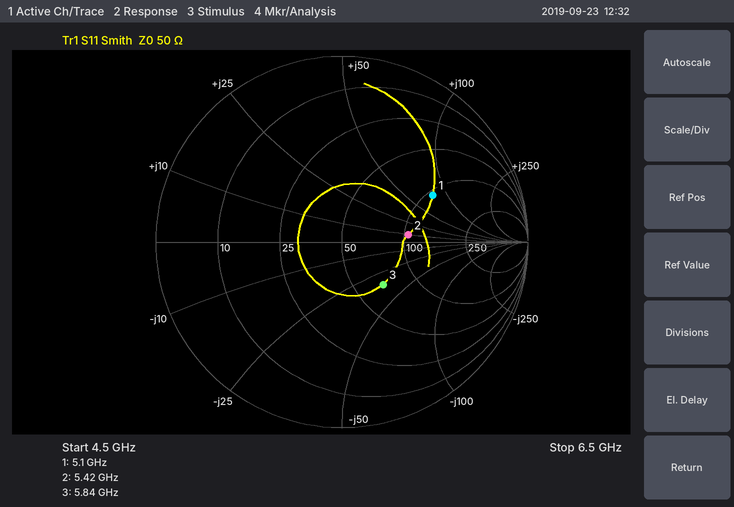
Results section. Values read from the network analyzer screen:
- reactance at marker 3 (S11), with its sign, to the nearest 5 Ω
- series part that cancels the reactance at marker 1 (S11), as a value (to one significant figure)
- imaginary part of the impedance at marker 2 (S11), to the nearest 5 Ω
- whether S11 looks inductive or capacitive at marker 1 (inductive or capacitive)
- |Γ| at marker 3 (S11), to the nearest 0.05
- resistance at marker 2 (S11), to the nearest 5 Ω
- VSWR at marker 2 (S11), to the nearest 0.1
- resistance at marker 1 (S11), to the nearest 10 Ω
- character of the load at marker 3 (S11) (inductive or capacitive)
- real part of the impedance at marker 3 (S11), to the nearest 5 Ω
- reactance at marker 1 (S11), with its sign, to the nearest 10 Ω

-35 Ω
400 fF
+10 Ω
inductive
0.30
105 Ω
2.1
110 Ω
capacitive
70 Ω
+80 Ω
